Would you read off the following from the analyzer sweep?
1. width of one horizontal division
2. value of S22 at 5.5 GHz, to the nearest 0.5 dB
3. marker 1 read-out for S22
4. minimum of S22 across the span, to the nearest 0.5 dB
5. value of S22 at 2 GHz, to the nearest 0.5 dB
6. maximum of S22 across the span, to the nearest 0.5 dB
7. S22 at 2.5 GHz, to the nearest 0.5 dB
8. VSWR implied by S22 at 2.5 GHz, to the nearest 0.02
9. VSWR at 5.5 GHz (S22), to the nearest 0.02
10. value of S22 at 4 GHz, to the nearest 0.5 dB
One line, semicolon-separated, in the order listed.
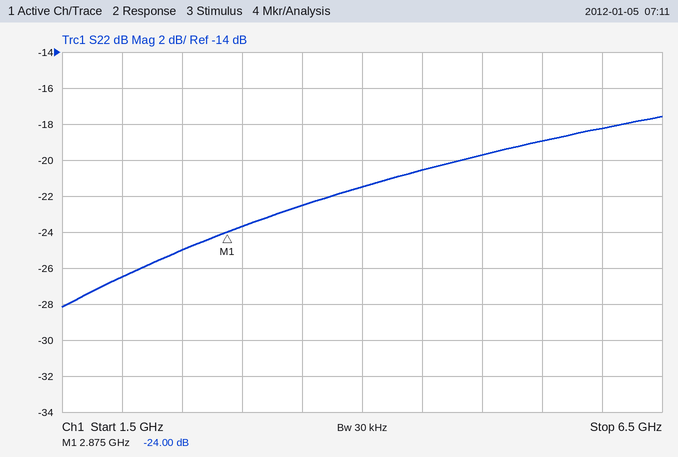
500 MHz; -19.0 dB; -24.00 dB; -28.0 dB; -26.5 dB; -17.5 dB; -25.0 dB; 1.12; 1.26; -21.5 dB
